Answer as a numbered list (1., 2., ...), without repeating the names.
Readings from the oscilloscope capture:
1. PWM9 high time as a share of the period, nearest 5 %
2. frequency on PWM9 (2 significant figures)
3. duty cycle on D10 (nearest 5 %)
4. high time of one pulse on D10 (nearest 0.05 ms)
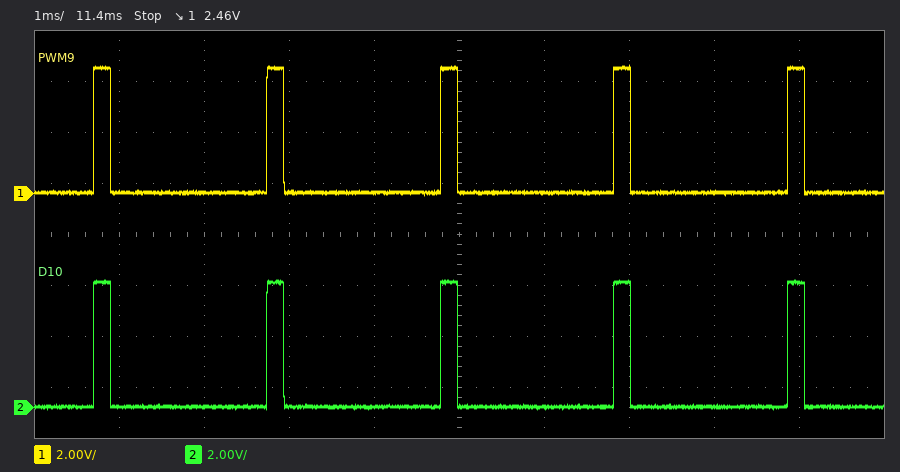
1. 10 %
2. 490 Hz
3. 10 %
4. 0.20 ms
